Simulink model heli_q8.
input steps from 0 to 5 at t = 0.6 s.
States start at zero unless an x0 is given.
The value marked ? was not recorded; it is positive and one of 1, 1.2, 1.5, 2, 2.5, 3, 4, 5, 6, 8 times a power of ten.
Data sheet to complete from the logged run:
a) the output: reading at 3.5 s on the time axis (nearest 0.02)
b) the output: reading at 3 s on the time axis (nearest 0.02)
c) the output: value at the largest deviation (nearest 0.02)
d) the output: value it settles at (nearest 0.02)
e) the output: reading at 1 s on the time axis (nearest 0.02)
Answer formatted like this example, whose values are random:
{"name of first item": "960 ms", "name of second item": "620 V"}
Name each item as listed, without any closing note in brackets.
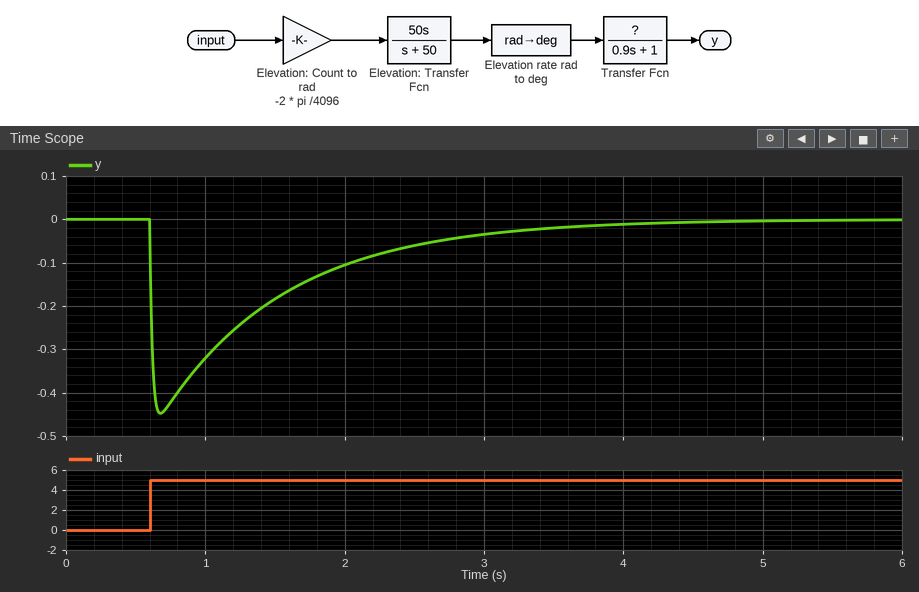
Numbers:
{"the output: reading at 3.5 s on the time axis": "-0.02", "the output: reading at 3 s on the time axis": "-0.04", "the output: value at the largest deviation": "-0.44", "the output: value it settles at": "0.00", "the output: reading at 1 s on the time axis": "-0.32"}
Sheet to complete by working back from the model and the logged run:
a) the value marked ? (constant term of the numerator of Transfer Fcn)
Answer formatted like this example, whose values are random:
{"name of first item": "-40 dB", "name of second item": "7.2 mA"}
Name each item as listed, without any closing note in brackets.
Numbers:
{"the value marked ?": "1"}
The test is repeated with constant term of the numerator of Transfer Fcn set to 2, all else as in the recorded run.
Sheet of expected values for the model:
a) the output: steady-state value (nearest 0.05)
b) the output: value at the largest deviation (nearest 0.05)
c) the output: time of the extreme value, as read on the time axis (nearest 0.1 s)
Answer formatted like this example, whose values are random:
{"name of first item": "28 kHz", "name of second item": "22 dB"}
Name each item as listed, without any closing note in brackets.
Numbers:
{"the output: steady-state value": "0.00", "the output: value at the largest deviation": "-0.90", "the output: time of the extreme value, as read on the time axis": "0.7 s"}
